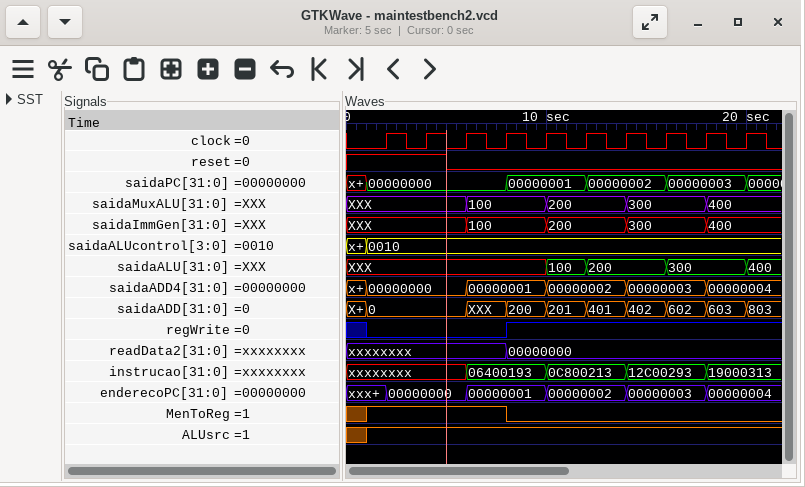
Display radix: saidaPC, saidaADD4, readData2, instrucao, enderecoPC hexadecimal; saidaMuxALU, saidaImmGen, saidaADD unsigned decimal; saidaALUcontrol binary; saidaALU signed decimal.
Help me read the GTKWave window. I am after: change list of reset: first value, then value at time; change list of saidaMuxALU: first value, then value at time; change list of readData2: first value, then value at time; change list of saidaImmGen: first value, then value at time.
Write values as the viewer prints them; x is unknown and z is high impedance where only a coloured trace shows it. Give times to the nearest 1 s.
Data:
1, 0 at 5 s
XXX, 100 at 6 s, 200 at 10 s, 300 at 14 s, 400 at 18 s
xxxxxxxx, 00000000 at 8 s
XXX, 100 at 6 s, 200 at 10 s, 300 at 14 s, 400 at 18 s
